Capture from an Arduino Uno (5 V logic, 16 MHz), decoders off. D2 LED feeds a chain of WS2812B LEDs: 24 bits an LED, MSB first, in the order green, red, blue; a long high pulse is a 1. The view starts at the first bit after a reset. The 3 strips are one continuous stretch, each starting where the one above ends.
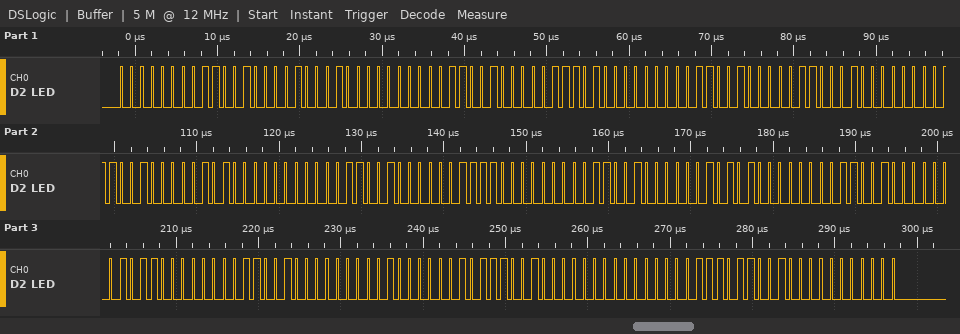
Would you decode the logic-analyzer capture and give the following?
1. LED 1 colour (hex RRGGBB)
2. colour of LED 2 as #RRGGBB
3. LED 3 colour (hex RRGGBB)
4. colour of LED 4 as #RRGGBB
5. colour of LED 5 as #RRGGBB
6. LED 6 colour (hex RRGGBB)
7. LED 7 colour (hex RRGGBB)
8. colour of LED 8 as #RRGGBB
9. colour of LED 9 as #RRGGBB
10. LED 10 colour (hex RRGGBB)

#C80044
#C8003A
#C80031
#C80028
#C8001E
#C80015
#C8000B
#C80002
#C80500
#C80E00
